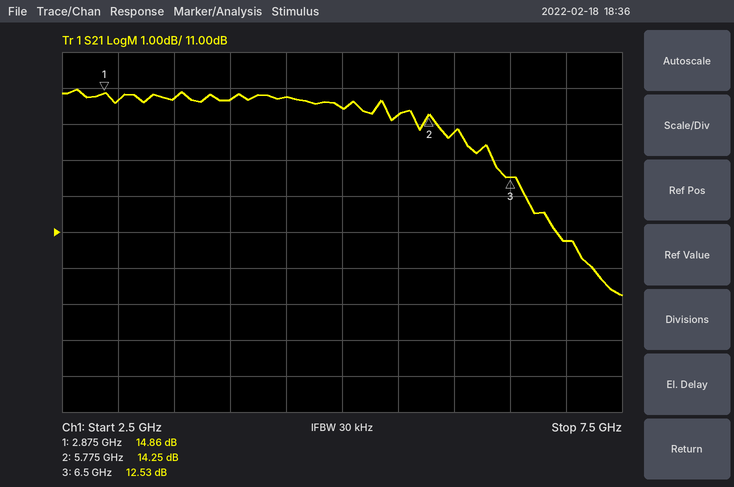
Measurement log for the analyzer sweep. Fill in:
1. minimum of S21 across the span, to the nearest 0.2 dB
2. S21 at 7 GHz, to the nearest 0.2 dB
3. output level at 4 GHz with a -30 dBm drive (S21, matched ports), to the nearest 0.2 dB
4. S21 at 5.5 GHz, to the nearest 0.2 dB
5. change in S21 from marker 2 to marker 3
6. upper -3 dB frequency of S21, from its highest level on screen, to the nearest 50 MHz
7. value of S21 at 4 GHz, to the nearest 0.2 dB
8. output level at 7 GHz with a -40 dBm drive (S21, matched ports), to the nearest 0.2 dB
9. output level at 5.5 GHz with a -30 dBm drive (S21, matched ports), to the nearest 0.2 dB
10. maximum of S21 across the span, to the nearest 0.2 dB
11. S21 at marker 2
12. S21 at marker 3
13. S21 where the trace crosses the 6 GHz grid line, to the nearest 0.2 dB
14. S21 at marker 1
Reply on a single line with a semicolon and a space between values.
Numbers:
9.2 dB; 10.8 dB; -15.4 dBm; 14.2 dB; -1.72 dB; 6.65 GHz; 14.6 dB; -29.2 dBm; -15.8 dBm; 15.0 dB; 14.25 dB; 12.53 dB; 13.8 dB; 14.86 dB
